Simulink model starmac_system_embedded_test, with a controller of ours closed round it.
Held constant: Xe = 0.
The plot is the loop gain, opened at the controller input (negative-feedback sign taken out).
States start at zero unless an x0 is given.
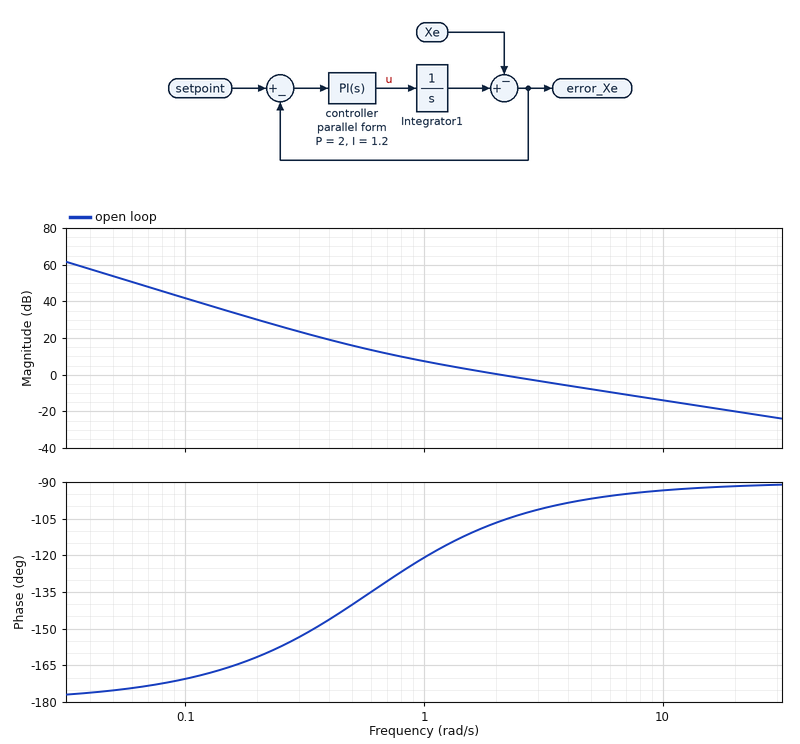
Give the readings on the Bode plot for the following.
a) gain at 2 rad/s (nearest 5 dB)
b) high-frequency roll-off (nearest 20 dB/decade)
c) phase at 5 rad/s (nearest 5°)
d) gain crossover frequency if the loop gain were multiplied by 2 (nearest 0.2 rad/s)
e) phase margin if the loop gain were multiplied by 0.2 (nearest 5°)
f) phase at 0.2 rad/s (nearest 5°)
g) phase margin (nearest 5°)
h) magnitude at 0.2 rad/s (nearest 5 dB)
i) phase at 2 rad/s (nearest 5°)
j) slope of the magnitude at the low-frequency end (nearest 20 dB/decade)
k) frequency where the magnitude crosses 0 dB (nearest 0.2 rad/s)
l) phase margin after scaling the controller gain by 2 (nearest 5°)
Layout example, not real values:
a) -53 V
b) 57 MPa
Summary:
a) 0 dB
b) -20 dB/decade
c) -95°
d) 4.0 rad/s
e) 45°
f) -160°
g) 75°
h) 30 dB
i) -105°
j) -40 dB/decade
k) 2.0 rad/s
l) 80°
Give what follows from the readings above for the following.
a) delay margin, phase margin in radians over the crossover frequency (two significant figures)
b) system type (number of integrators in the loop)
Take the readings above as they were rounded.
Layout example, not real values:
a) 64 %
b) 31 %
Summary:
a) 0.65 s
b) 2
